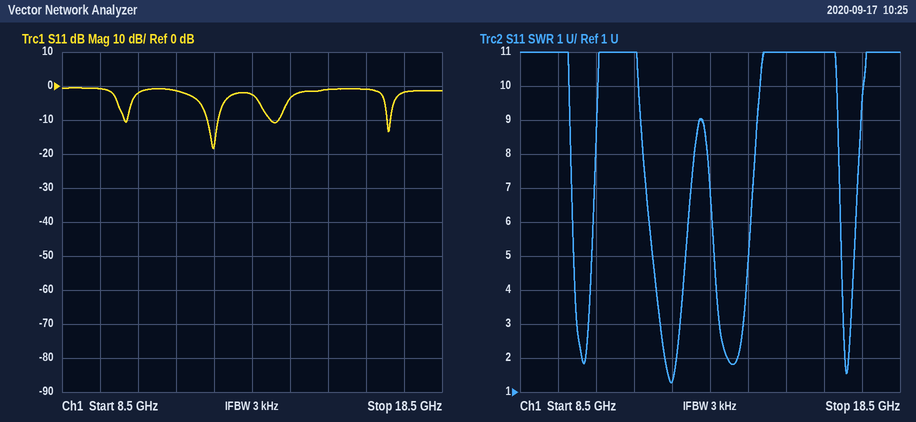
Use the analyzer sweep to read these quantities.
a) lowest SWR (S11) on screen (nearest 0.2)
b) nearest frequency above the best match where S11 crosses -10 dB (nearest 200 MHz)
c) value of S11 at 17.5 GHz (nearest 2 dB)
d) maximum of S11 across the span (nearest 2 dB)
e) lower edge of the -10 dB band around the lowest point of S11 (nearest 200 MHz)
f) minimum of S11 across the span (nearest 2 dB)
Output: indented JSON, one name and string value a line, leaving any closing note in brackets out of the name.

{
  "lowest SWR (S11) on screen": "1.2",
  "nearest frequency above the best match where S11 crosses -10 dB": "12.6 GHz",
  "value of S11 at 17.5 GHz": "-2 dB",
  "maximum of S11 across the span": "0 dB",
  "lower edge of the -10 dB band around the lowest point of S11": "12.4 GHz",
  "minimum of S11 across the span": "-18 dB"
}
